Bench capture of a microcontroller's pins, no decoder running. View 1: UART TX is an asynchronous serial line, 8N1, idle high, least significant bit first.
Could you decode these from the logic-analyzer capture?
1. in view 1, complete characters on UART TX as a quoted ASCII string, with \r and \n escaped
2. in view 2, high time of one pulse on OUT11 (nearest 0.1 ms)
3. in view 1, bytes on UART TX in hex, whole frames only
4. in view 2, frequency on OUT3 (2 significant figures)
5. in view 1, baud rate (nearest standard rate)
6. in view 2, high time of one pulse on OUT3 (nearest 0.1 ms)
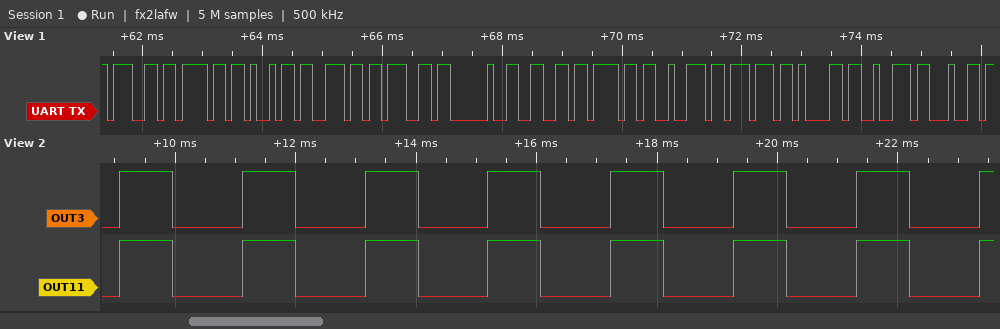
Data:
"going forward"
0.9 ms
0x67 0x6F 0x69 0x6E 0x67 0x20 0x66 0x6F 0x72 0x77 0x61 0x72 0x64
490 Hz
9600 baud
0.9 ms
